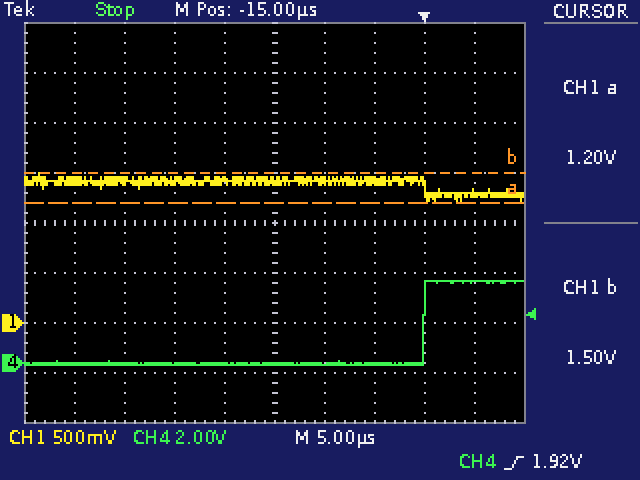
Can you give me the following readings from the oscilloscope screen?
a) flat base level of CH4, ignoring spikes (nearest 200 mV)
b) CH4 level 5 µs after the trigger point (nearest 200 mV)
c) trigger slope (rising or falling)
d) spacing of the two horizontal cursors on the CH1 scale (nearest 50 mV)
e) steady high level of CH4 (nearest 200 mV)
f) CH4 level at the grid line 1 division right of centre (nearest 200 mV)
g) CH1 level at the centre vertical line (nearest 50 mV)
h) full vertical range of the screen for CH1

0.0 V
3.2 V
rising
300 mV
3.2 V
0.0 V
1.40 V
4 V
